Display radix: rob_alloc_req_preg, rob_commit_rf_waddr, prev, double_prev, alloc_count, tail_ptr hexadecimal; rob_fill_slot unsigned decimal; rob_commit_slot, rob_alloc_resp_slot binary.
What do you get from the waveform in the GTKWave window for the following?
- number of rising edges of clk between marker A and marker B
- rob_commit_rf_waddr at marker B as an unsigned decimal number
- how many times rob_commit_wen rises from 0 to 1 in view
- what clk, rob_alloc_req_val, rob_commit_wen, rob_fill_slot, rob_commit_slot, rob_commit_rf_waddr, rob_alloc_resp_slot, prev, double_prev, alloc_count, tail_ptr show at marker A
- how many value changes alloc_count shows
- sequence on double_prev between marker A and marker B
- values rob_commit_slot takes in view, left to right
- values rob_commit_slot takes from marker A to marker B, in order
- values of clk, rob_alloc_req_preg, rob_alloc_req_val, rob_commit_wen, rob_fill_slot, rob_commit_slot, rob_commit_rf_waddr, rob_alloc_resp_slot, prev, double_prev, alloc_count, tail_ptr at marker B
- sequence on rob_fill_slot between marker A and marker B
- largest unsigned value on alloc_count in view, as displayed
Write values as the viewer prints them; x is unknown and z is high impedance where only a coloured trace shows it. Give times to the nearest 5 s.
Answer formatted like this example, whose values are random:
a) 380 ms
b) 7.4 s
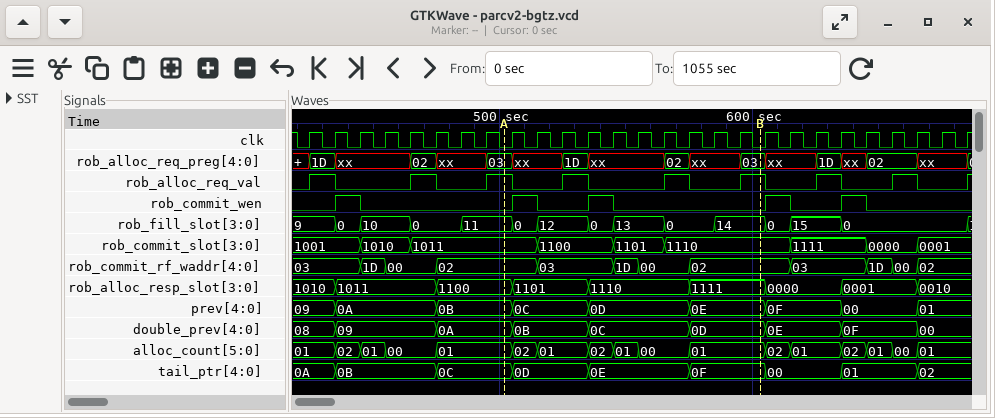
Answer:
a) 10
b) 2
c) 5
d) clk=0, rob_alloc_req_val=1, rob_commit_wen=0, rob_fill_slot=11, rob_commit_slot=1011, rob_commit_rf_waddr=02, rob_alloc_resp_slot=1100, prev=0B, double_prev=0A, alloc_count=01, tail_ptr=0C
e) 16
f) 0A, 0B, 0C, 0D
g) 1001, 1010, 1011, 1100, 1101, 1110, 1111, 0000, 0001
h) 1011, 1100, 1101, 1110
i) clk=0, rob_alloc_req_preg=03, rob_alloc_req_val=1, rob_commit_wen=0, rob_fill_slot=14, rob_commit_slot=1110, rob_commit_rf_waddr=02, rob_alloc_resp_slot=1111, prev=0E, double_prev=0D, alloc_count=01, tail_ptr=0F
j) 11, 0, 12, 0, 13, 0, 14
k) 02
